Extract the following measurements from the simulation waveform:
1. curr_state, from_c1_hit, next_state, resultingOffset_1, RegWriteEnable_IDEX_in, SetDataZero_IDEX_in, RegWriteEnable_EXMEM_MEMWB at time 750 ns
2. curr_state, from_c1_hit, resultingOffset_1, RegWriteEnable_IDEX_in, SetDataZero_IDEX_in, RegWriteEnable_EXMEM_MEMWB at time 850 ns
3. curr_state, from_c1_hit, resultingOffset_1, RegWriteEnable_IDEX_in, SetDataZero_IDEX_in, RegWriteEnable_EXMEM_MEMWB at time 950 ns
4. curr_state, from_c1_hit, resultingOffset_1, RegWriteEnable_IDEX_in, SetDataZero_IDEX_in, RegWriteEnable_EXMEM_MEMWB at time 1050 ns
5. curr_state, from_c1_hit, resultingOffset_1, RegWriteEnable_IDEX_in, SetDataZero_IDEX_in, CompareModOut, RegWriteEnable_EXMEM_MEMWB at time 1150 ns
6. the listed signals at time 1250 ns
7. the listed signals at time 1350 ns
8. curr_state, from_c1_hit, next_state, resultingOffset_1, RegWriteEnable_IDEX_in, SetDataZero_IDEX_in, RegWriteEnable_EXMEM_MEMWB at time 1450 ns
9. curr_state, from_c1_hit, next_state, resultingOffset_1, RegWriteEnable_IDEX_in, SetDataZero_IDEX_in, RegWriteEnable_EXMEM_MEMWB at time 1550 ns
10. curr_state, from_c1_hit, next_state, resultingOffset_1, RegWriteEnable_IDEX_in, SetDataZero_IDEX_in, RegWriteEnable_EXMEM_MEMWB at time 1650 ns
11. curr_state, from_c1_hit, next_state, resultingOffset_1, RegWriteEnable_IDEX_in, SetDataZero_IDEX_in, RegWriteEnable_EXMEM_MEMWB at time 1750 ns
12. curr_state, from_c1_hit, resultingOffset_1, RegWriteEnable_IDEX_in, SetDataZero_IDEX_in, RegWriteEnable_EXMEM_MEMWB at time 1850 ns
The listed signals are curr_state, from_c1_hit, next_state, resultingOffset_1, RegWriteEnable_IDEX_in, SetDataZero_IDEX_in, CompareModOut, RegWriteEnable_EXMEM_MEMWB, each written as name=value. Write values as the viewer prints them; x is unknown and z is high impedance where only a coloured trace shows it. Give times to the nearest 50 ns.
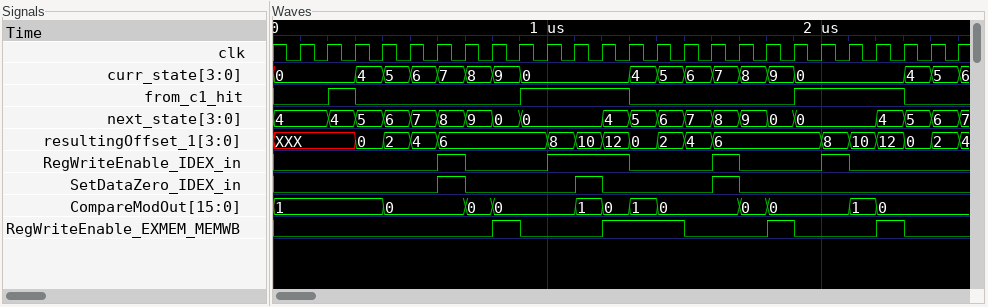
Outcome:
curr_state=8, from_c1_hit=0, next_state=9, resultingOffset_1=6, RegWriteEnable_IDEX_in=0, SetDataZero_IDEX_in=0, RegWriteEnable_EXMEM_MEMWB=0
curr_state=9, from_c1_hit=0, resultingOffset_1=6, RegWriteEnable_IDEX_in=0, SetDataZero_IDEX_in=0, RegWriteEnable_EXMEM_MEMWB=1
curr_state=0, from_c1_hit=1, resultingOffset_1=6, RegWriteEnable_IDEX_in=0, SetDataZero_IDEX_in=0, RegWriteEnable_EXMEM_MEMWB=0
curr_state=0, from_c1_hit=1, resultingOffset_1=8, RegWriteEnable_IDEX_in=1, SetDataZero_IDEX_in=0, RegWriteEnable_EXMEM_MEMWB=0
curr_state=0, from_c1_hit=1, resultingOffset_1=10, RegWriteEnable_IDEX_in=1, SetDataZero_IDEX_in=1, CompareModOut=1, RegWriteEnable_EXMEM_MEMWB=0
curr_state=0, from_c1_hit=1, next_state=4, resultingOffset_1=12, RegWriteEnable_IDEX_in=1, SetDataZero_IDEX_in=0, CompareModOut=0, RegWriteEnable_EXMEM_MEMWB=1
curr_state=4, from_c1_hit=0, next_state=5, resultingOffset_1=0, RegWriteEnable_IDEX_in=0, SetDataZero_IDEX_in=0, CompareModOut=1, RegWriteEnable_EXMEM_MEMWB=1
curr_state=5, from_c1_hit=0, next_state=6, resultingOffset_1=2, RegWriteEnable_IDEX_in=0, SetDataZero_IDEX_in=0, RegWriteEnable_EXMEM_MEMWB=1
curr_state=6, from_c1_hit=0, next_state=7, resultingOffset_1=4, RegWriteEnable_IDEX_in=0, SetDataZero_IDEX_in=0, RegWriteEnable_EXMEM_MEMWB=0
curr_state=7, from_c1_hit=0, next_state=8, resultingOffset_1=6, RegWriteEnable_IDEX_in=1, SetDataZero_IDEX_in=1, RegWriteEnable_EXMEM_MEMWB=0
curr_state=8, from_c1_hit=0, next_state=9, resultingOffset_1=6, RegWriteEnable_IDEX_in=0, SetDataZero_IDEX_in=0, RegWriteEnable_EXMEM_MEMWB=0
curr_state=9, from_c1_hit=0, resultingOffset_1=6, RegWriteEnable_IDEX_in=0, SetDataZero_IDEX_in=0, RegWriteEnable_EXMEM_MEMWB=1
